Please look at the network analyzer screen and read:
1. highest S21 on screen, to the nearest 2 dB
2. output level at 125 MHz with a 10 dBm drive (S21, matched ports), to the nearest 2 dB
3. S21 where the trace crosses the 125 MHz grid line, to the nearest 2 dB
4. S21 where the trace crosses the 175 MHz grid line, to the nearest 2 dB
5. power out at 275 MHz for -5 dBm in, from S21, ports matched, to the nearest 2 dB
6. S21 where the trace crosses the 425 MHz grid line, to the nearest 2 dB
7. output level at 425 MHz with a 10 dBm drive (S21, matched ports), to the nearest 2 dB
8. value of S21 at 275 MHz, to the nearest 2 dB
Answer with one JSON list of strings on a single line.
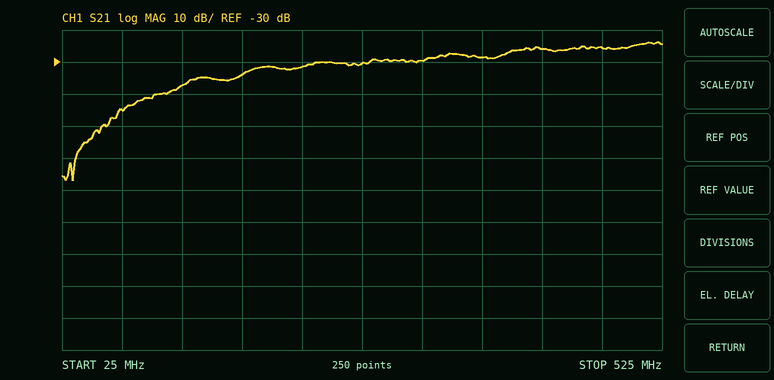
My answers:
["-24 dB", "-28 dBm", "-38 dB", "-34 dB", "-36 dBm", "-26 dB", "-16 dBm", "-30 dB"]
